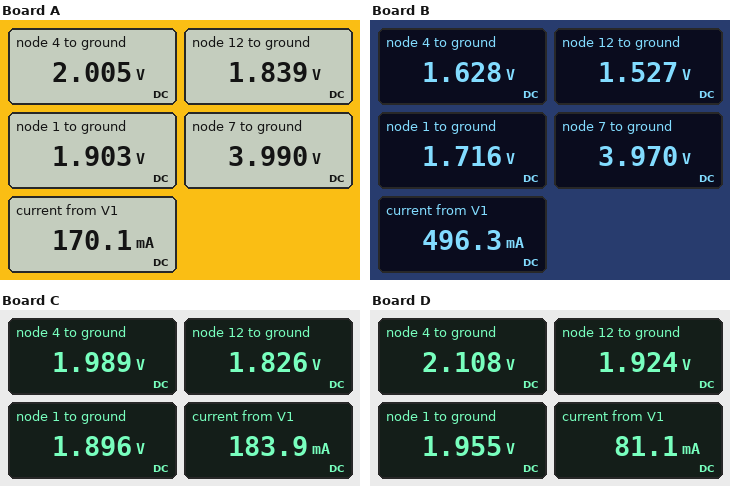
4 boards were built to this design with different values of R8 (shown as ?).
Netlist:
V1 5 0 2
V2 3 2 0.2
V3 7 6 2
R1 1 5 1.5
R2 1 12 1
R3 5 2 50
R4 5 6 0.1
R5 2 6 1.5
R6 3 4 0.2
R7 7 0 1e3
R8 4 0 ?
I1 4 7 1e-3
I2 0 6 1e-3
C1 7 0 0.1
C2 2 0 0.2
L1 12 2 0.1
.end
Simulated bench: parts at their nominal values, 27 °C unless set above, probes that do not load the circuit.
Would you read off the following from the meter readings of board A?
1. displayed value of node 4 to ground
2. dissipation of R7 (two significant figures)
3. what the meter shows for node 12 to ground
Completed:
2.005 V
16 mW
1.839 V
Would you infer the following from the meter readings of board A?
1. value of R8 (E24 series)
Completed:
12 Ω
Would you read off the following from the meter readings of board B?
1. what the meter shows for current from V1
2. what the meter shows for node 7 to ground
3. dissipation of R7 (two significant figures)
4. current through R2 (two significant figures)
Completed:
496.3 mA
3.970 V
16 mW
190 mA
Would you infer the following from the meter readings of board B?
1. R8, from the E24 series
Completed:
3.3 Ω
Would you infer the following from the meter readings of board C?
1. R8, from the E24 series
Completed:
11 Ω
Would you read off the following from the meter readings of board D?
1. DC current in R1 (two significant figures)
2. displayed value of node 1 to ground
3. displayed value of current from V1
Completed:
30 mA
1.955 V
81.1 mA
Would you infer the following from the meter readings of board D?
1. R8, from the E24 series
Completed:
27 Ω
